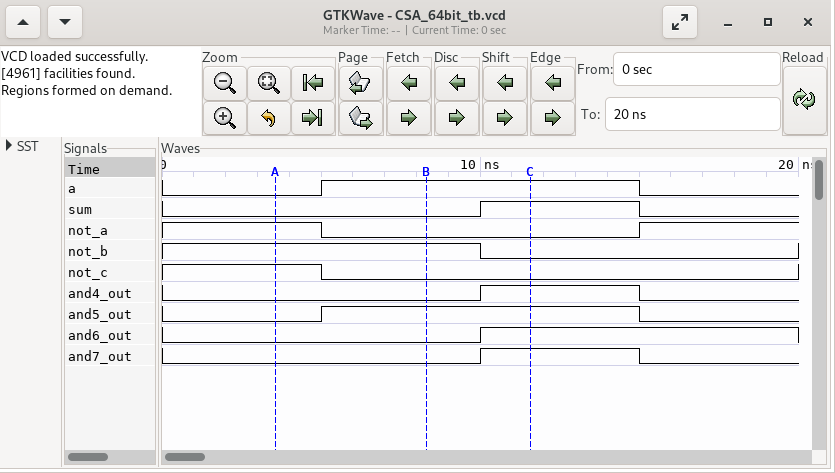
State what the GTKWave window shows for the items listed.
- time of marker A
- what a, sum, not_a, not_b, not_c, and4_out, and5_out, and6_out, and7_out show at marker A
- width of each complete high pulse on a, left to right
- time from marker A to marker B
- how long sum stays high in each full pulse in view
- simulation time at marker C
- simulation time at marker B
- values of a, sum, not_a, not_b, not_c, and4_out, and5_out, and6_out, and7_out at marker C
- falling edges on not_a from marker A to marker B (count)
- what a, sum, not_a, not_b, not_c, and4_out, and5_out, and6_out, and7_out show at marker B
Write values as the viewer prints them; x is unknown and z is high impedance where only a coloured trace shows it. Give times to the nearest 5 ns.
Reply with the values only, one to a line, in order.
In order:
5 ns
a=0, sum=0, not_a=1, not_b=1, not_c=1, and4_out=0, and5_out=0, and6_out=0, and7_out=0
10 ns
5 ns
5 ns
10 ns
10 ns
a=1, sum=1, not_a=0, not_b=0, not_c=0, and4_out=1, and5_out=1, and6_out=1, and7_out=1
1
a=1, sum=0, not_a=0, not_b=1, not_c=0, and4_out=0, and5_out=1, and6_out=0, and7_out=0
